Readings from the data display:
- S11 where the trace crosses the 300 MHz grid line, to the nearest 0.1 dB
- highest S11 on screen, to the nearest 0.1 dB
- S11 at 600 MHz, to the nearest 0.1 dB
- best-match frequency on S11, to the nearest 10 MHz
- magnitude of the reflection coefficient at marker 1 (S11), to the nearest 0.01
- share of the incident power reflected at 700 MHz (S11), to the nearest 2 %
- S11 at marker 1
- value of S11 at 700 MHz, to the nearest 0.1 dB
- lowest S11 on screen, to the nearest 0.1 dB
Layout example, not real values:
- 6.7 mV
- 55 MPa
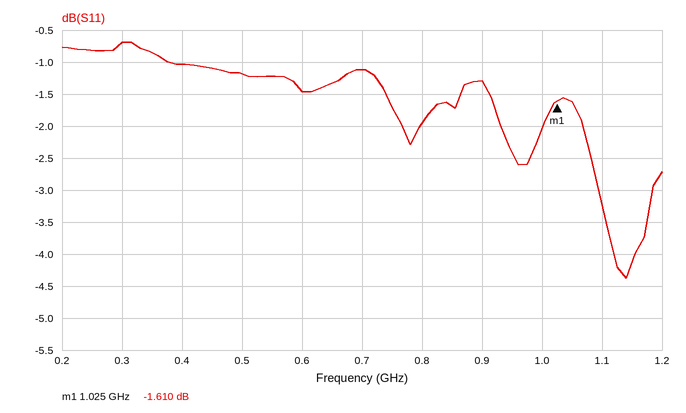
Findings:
- -0.7 dB
- -0.7 dB
- -1.5 dB
- 1.14 GHz
- 0.83
- 78 %
- -1.610 dB
- -1.1 dB
- -4.4 dB
